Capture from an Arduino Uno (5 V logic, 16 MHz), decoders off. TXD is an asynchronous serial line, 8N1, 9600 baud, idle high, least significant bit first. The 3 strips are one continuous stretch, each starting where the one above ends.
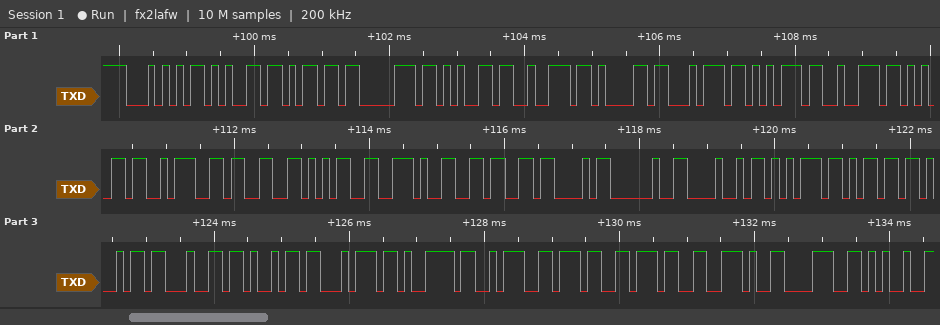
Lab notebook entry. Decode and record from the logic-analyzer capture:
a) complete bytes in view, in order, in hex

54 65 6D 70 65 72 61 74 75 72 65 3A 33 35 2E 36 43 20 48 75 6D 69 64 69 74 79 3A 37 37 2E 38 25
